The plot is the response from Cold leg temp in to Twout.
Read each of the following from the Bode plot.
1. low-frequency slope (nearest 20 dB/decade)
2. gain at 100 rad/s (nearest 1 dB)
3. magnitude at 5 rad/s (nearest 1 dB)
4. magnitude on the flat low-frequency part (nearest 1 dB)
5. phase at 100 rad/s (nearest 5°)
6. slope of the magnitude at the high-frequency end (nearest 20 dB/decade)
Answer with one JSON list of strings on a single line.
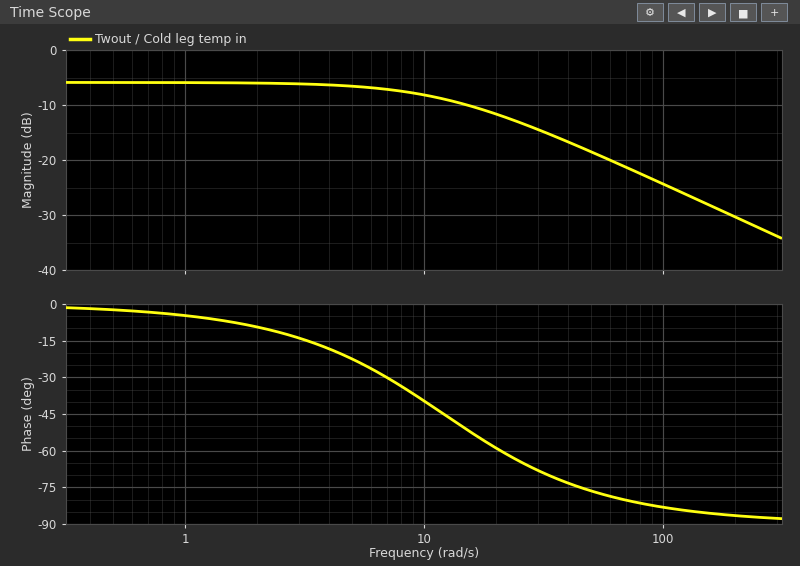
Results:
["0 dB/decade", "-24 dB", "-7 dB", "-6 dB", "-85°", "-20 dB/decade"]
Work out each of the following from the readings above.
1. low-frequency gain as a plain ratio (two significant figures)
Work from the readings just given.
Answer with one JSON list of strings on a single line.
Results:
["0.50"]
